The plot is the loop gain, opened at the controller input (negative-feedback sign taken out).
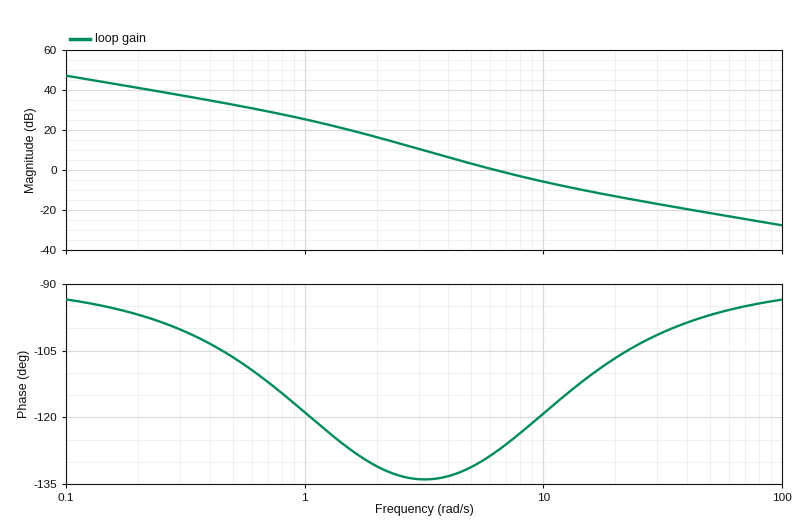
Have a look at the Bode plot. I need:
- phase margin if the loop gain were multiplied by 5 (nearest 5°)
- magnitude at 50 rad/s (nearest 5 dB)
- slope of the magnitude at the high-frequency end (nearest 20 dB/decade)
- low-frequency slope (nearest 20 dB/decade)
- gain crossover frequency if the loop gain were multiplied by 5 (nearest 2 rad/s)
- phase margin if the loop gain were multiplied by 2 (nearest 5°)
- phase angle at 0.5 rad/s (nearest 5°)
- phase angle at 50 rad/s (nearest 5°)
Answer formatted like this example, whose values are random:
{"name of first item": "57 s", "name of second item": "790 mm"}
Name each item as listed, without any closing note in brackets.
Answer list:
{"phase margin if the loop gain were multiplied by 5": "75°", "magnitude at 50 rad/s": "-20 dB", "slope of the magnitude at the high-frequency end": "-20 dB/decade", "low-frequency slope": "-20 dB/decade", "gain crossover frequency if the loop gain were multiplied by 5": "22 rad/s", "phase margin if the loop gain were multiplied by 2": "60°", "phase angle at 0.5 rad/s": "-105°", "phase angle at 50 rad/s": "-95°"}
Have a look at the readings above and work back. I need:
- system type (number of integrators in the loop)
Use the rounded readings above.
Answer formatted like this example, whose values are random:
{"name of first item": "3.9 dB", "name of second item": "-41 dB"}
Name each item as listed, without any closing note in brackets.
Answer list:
{"system type": "1"}
